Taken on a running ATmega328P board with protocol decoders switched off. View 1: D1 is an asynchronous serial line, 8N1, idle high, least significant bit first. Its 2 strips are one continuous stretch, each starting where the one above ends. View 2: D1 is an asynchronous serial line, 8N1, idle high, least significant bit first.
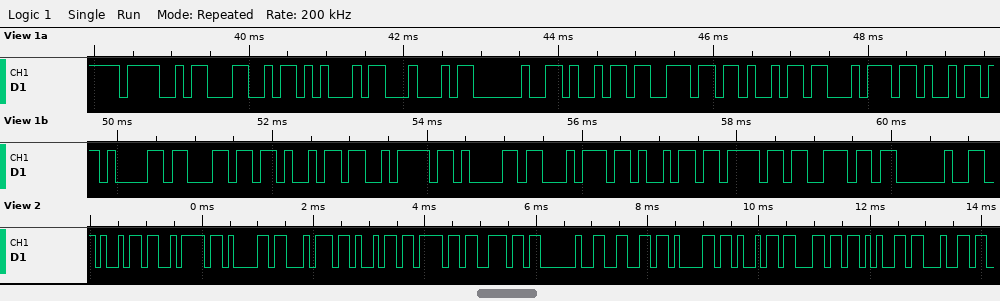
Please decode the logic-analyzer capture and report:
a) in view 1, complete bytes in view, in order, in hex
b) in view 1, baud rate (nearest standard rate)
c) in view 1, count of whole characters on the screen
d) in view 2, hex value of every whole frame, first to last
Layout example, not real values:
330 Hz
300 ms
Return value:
4F 4C 45 44 20 69 6E 69 74 69 61 6C 69 7A 61 74 69 6F 6E 20
9600 baud
20
0x69 0x7A 0x61 0x74 0x69 0x6F 0x6E 0x20 0x66 0x61 0x69 0x6C 0x65 0x64
